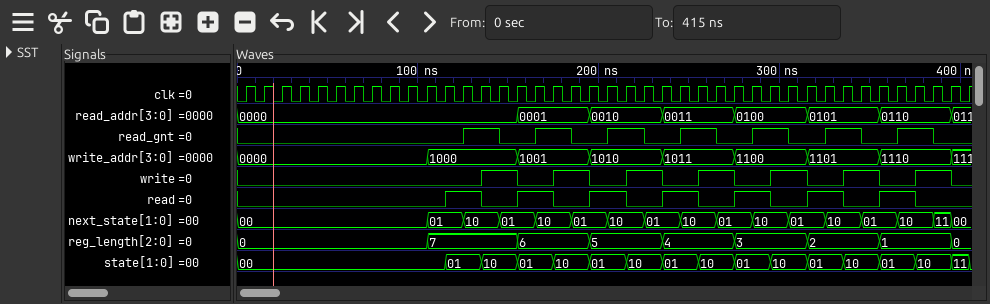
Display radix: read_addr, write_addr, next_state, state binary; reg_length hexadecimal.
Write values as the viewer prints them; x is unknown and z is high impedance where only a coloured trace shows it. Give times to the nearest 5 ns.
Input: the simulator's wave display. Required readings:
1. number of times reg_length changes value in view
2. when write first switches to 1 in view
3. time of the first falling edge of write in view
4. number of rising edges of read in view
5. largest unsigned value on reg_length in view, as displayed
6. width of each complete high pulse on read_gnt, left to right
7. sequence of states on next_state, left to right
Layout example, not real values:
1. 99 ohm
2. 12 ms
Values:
1. 8
2. 135 ns
3. 155 ns
4. 7
5. 7
6. 20 ns, 20 ns, 20 ns, 20 ns, 20 ns, 20 ns, 20 ns
7. 00, 01, 10, 01, 10, 01, 10, 01, 10, 01, 10, 01, 10, 01, 10, 11, 00
